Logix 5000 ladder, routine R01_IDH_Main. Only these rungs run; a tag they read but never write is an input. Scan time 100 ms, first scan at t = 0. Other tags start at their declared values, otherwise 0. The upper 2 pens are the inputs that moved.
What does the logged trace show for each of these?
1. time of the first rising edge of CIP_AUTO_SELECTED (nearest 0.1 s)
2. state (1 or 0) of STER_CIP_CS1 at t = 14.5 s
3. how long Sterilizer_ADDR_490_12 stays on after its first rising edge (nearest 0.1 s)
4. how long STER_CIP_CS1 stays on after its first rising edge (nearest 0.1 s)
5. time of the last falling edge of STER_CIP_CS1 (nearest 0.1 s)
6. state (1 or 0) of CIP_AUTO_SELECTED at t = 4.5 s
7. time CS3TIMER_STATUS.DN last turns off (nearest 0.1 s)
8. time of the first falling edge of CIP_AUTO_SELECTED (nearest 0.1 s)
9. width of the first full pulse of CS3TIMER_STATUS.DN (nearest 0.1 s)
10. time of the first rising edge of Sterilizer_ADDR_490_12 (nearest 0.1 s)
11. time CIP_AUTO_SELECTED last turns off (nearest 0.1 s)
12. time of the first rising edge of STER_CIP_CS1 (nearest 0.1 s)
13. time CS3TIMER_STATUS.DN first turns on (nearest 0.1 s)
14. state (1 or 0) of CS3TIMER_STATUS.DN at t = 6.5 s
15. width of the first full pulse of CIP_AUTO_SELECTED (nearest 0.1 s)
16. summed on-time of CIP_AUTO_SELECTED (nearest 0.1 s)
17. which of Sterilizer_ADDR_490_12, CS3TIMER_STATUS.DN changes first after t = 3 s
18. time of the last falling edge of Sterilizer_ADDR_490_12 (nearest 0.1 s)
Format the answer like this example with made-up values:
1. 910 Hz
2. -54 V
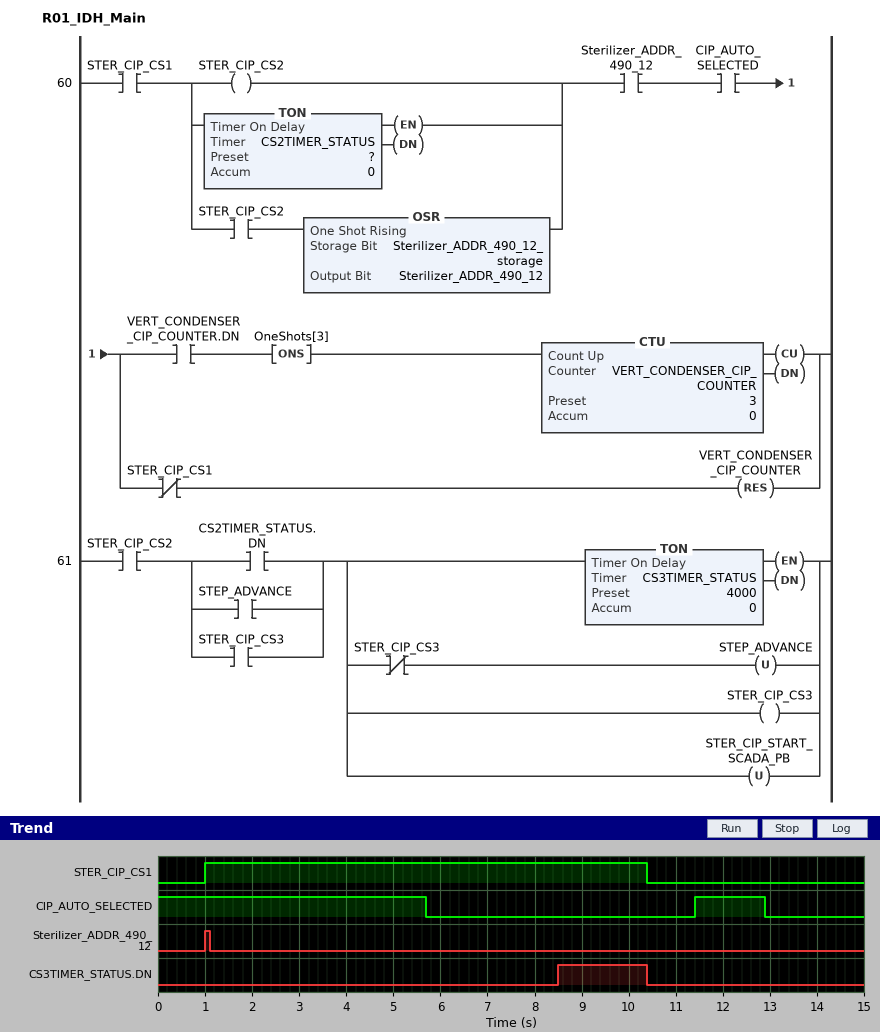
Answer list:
1. 11.4 s
2. 0
3. 0.1 s
4. 9.4 s
5. 10.4 s
6. 1
7. 10.4 s
8. 5.7 s
9. 1.9 s
10. 1.0 s
11. 12.9 s
12. 1.0 s
13. 8.5 s
14. 0
15. 1.5 s
16. 7.2 s
17. CS3TIMER_STATUS.DN
18. 1.1 s
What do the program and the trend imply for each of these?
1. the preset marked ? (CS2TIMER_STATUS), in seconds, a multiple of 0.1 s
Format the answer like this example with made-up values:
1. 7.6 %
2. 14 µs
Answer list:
1. 3.5 s
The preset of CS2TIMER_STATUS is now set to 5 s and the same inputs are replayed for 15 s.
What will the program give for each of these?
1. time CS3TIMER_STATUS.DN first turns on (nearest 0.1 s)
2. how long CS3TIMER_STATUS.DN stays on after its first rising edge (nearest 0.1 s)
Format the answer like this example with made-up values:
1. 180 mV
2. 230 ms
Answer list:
1. 10.0 s
2. 0.4 s
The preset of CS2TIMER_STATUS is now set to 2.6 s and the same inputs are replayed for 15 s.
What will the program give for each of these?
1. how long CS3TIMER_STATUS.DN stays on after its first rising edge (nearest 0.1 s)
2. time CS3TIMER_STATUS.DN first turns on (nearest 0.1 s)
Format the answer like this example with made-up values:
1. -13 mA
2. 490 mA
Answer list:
1. 2.8 s
2. 7.6 s
